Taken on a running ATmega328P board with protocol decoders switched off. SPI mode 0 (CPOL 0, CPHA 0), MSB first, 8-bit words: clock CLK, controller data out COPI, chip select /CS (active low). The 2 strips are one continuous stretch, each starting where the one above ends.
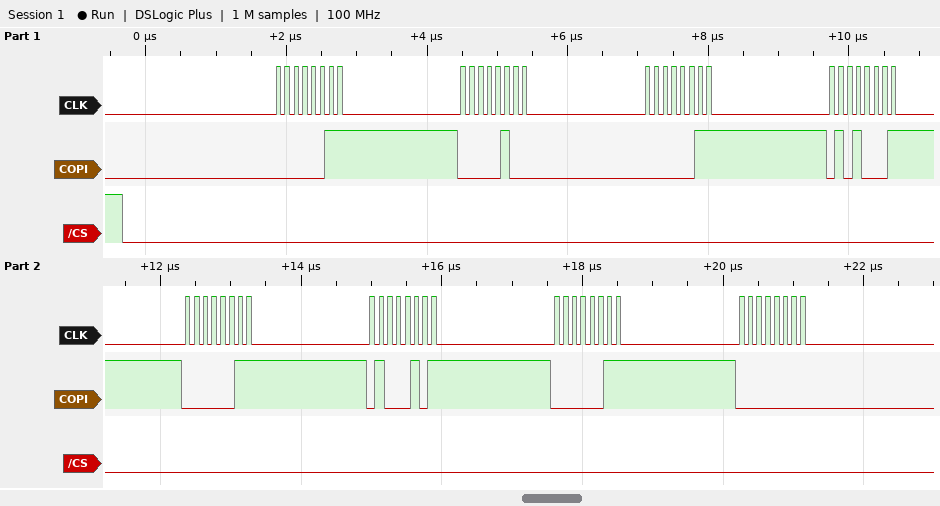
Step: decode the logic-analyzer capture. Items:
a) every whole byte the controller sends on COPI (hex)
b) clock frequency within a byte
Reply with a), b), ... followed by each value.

a) 0x03 0x04 0x03 0x51 0x03 0x45 0x03 0x00
b) 8 MHz
